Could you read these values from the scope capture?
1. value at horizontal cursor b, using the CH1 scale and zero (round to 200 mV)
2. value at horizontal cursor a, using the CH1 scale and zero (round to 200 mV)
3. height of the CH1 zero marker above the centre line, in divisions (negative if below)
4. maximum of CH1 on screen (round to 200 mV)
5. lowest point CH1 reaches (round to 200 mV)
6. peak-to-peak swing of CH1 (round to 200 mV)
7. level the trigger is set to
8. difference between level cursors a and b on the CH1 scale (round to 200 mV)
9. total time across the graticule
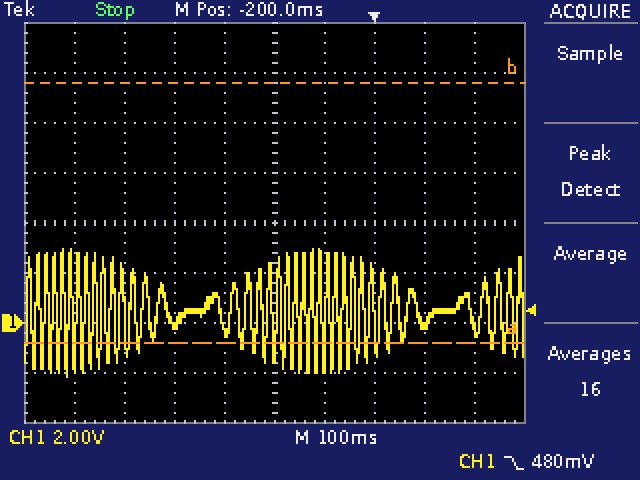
9.6 V
-800 mV
-2.0 div
3.0 V
-2.2 V
5.2 V
480 mV
10.4 V
1 s
